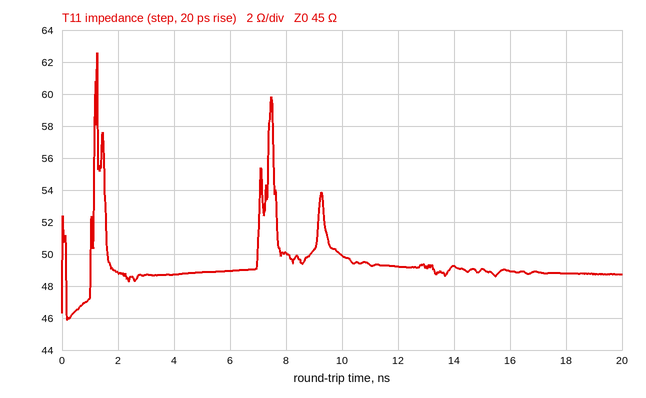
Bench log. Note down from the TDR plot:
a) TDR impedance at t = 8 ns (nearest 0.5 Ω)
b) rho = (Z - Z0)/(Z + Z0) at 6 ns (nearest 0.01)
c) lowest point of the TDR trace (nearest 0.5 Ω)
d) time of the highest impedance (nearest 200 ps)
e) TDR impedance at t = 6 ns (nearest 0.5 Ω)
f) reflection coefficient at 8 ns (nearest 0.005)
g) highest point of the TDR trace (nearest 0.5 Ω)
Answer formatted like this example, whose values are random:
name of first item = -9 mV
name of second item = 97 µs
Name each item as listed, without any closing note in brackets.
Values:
TDR impedance at t = 8 ns = 50.0 Ω
rho = (Z - Z0)/(Z + Z0) at 6 ns = +0.04
lowest point of the TDR trace = 46.0 Ω
time of the highest impedance = 1.2 ns
TDR impedance at t = 6 ns = 49.0 Ω
reflection coefficient at 8 ns = +0.055
highest point of the TDR trace = 62.5 Ω
